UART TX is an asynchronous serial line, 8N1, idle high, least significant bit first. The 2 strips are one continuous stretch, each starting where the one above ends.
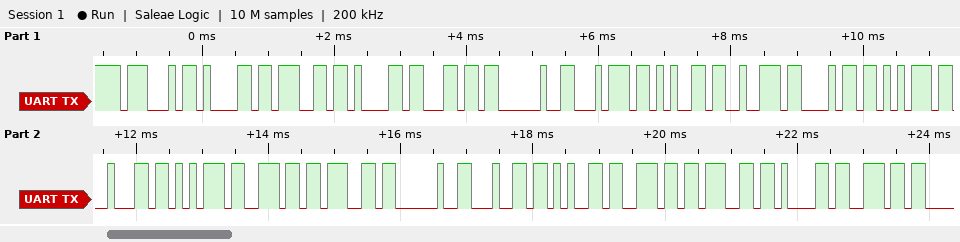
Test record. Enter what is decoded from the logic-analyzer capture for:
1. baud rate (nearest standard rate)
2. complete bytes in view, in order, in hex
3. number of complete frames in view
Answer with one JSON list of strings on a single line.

["9600 baud", "47 61 67 61 6C 20 74 65 72 68 75 62 75 6E 67 20 64 65 6E 67 61 6E", "22"]
